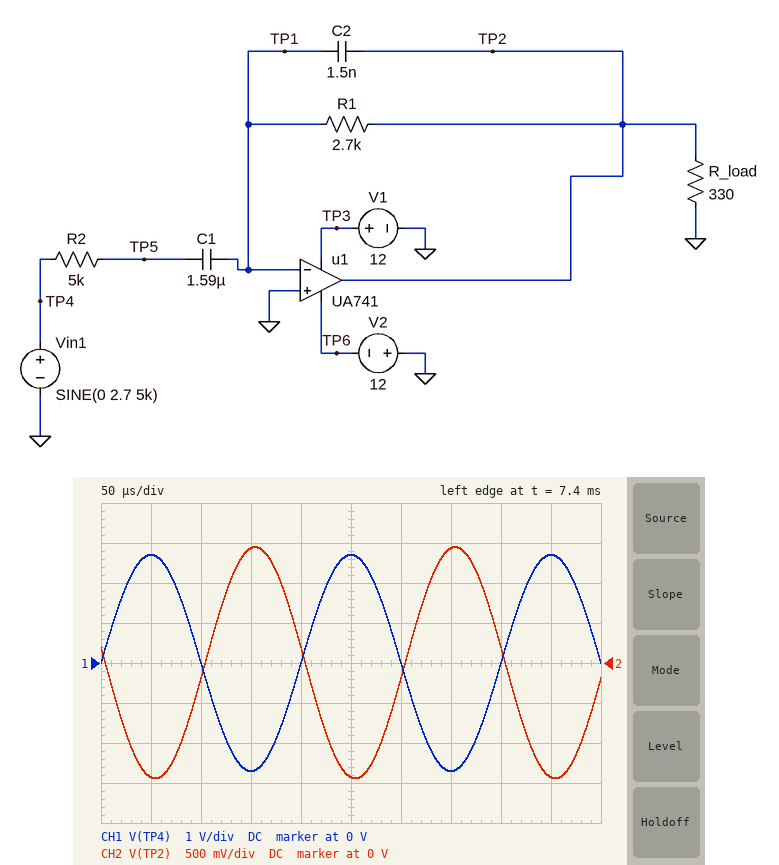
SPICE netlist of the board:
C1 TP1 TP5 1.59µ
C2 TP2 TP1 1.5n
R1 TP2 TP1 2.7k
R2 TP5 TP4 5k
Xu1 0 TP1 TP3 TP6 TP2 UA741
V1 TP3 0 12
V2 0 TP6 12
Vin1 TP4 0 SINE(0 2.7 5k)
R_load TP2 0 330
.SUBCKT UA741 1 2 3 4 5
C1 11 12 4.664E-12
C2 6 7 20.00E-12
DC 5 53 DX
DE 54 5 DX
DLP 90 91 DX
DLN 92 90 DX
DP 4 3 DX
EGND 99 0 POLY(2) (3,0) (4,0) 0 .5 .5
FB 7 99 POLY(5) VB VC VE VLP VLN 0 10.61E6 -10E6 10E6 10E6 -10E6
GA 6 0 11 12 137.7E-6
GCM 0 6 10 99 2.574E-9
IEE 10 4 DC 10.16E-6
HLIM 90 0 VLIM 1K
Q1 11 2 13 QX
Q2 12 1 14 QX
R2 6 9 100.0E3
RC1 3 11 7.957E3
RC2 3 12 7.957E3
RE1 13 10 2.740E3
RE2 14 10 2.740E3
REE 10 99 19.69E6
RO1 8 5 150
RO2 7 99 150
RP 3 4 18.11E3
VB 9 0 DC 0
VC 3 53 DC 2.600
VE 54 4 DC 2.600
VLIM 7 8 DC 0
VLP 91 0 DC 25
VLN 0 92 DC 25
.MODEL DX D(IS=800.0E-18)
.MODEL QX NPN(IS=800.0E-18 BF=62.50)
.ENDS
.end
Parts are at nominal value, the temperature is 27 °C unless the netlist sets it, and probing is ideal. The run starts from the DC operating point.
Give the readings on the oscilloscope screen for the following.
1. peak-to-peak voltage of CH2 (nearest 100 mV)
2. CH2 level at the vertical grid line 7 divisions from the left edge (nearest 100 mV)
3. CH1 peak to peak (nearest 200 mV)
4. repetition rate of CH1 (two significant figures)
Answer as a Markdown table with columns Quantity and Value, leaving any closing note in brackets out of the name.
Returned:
| Quantity | Value |
|---|---|
| peak-to-peak voltage of CH2 | 2.9 V |
| CH2 level at the vertical grid line 7 divisions from the left edge | 1.4 V |
| CH1 peak to peak | 5.4 V |
| repetition rate of CH1 | 5.0 kHz |
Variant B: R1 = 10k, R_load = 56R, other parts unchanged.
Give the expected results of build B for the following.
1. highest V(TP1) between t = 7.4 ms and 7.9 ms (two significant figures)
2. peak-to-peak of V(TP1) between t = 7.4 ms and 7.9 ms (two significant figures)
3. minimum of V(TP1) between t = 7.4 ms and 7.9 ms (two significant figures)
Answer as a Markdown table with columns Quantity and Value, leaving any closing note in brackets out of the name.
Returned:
| Quantity | Value |
|---|---|
| highest V(TP1) between t = 7.4 ms and 7.9 ms | 1.3 V |
| peak-to-peak of V(TP1) between t = 7.4 ms and 7.9 ms | 2.6 V |
| minimum of V(TP1) between t = 7.4 ms and 7.9 ms | -1.3 V |
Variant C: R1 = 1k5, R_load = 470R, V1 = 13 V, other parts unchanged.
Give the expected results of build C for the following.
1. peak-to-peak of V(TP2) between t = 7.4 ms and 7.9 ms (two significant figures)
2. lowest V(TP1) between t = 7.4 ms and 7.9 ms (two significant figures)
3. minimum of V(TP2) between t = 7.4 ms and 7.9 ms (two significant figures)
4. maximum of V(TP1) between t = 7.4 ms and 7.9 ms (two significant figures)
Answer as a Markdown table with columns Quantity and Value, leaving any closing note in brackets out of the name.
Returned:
| Quantity | Value |
|---|---|
| peak-to-peak of V(TP2) between t = 7.4 ms and 7.9 ms | 1.6 V |
| lowest V(TP1) between t = 7.4 ms and 7.9 ms | -5.2 mV |
| minimum of V(TP2) between t = 7.4 ms and 7.9 ms | -810 mV |
| maximum of V(TP1) between t = 7.4 ms and 7.9 ms | 5.3 mV |
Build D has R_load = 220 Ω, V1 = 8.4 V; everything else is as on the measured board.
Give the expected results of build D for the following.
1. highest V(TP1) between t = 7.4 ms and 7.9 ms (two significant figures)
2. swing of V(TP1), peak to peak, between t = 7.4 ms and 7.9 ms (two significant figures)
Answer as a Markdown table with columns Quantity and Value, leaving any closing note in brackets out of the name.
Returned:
| Quantity | Value |
|---|---|
| highest V(TP1) between t = 7.4 ms and 7.9 ms | 11 mV |
| swing of V(TP1), peak to peak, between t = 7.4 ms and 7.9 ms | 23 mV |
